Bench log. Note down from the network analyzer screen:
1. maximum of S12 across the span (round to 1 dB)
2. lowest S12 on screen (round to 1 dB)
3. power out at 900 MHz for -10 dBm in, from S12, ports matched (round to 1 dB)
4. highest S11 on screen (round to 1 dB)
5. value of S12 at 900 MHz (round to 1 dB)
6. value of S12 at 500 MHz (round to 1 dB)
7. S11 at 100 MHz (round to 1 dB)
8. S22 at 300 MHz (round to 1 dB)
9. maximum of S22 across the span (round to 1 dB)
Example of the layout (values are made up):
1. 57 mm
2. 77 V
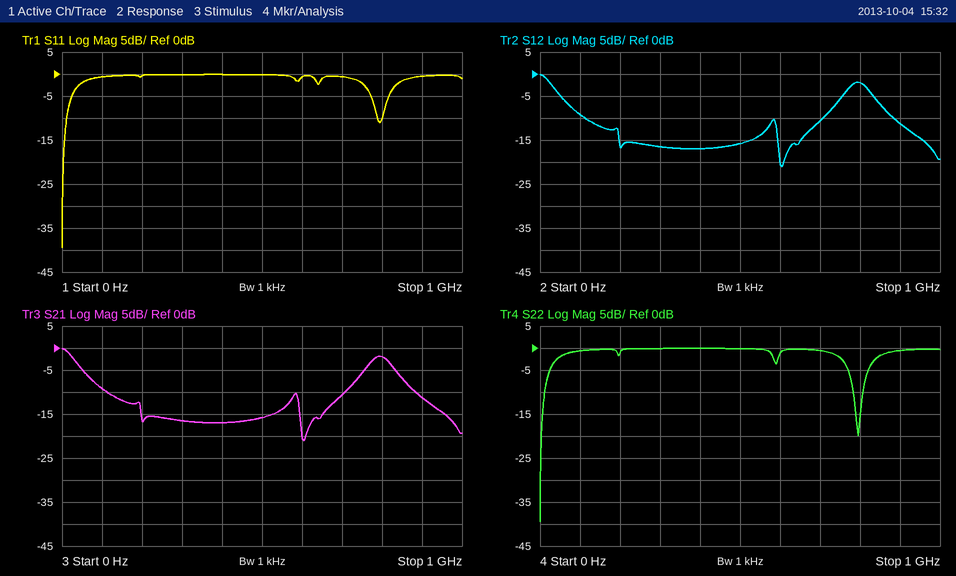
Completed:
1. 0 dB
2. -21 dB
3. -21 dBm
4. 0 dB
5. -11 dB
6. -16 dB
7. -1 dB
8. 0 dB
9. 0 dB
